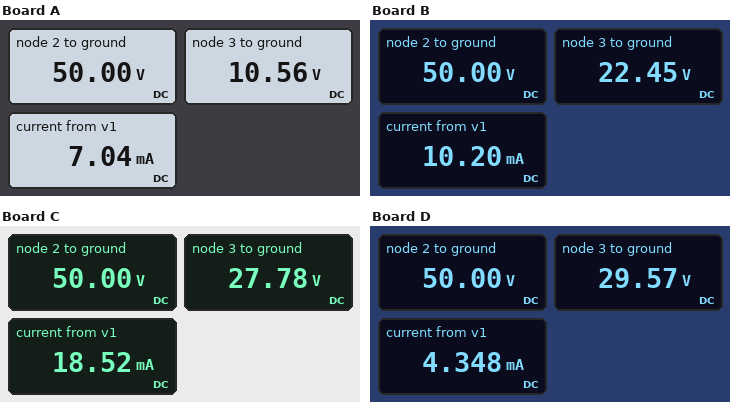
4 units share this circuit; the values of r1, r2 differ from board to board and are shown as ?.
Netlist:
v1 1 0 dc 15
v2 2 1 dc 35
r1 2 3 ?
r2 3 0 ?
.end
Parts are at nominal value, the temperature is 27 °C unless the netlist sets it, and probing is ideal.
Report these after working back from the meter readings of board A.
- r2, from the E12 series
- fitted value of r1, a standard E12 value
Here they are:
1.5 kΩ
5.6 kΩ
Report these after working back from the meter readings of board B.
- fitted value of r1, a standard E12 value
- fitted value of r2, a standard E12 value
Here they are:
2.7 kΩ
2.2 kΩ
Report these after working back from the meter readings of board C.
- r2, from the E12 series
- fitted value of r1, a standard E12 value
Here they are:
1.5 kΩ
1.2 kΩ
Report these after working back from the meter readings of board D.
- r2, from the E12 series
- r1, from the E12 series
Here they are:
6.8 kΩ
4.7 kΩ
